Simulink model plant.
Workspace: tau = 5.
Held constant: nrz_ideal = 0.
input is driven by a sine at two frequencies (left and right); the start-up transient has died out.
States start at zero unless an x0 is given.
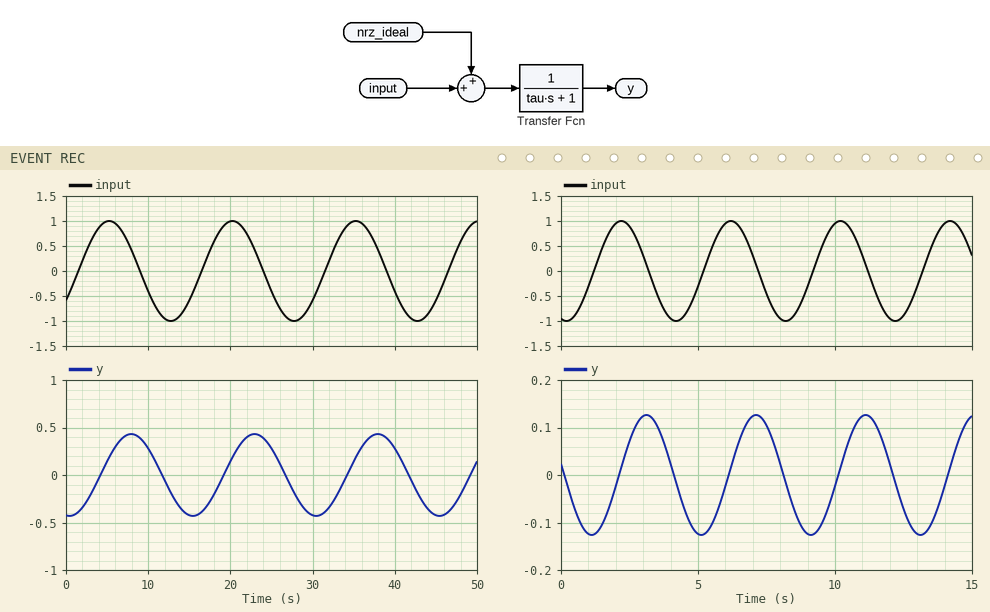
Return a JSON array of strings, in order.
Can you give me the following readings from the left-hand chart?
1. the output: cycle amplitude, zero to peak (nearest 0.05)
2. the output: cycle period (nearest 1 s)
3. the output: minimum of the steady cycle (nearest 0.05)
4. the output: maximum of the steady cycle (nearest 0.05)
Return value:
["0.45", "15 s", "-0.45", "0.45"]
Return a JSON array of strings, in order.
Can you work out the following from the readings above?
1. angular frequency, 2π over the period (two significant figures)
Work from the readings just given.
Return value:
["0.42 rad/s"]
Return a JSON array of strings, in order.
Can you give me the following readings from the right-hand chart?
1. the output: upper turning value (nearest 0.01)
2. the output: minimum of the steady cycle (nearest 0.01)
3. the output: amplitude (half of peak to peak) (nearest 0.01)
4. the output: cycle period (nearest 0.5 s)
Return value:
["0.13", "-0.13", "0.13", "4.0 s"]
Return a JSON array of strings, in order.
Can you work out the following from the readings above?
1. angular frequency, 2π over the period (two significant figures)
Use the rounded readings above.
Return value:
["1.6 rad/s"]
